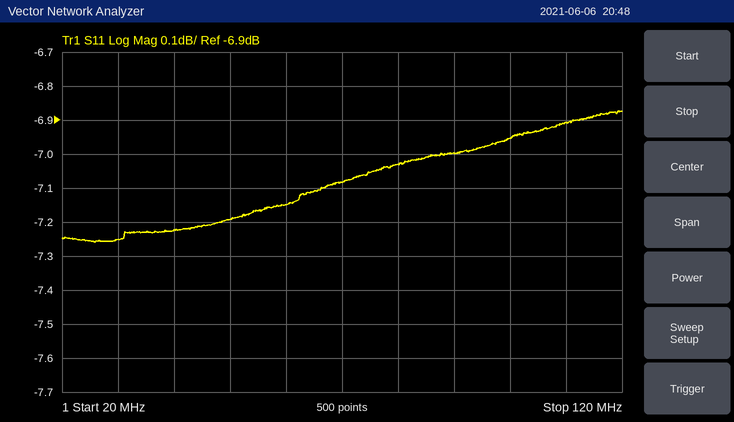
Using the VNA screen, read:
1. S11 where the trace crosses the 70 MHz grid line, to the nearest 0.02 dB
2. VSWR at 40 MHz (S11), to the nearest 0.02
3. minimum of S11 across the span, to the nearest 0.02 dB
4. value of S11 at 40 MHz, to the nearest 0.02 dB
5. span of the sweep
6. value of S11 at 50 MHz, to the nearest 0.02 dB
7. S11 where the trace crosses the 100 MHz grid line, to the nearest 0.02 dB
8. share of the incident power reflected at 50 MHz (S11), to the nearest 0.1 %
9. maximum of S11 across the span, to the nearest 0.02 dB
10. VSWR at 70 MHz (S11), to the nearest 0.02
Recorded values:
-7.08 dB
2.54
-7.26 dB
-7.22 dB
100 MHz
-7.20 dB
-6.96 dB
19.1 %
-6.88 dB
2.58
